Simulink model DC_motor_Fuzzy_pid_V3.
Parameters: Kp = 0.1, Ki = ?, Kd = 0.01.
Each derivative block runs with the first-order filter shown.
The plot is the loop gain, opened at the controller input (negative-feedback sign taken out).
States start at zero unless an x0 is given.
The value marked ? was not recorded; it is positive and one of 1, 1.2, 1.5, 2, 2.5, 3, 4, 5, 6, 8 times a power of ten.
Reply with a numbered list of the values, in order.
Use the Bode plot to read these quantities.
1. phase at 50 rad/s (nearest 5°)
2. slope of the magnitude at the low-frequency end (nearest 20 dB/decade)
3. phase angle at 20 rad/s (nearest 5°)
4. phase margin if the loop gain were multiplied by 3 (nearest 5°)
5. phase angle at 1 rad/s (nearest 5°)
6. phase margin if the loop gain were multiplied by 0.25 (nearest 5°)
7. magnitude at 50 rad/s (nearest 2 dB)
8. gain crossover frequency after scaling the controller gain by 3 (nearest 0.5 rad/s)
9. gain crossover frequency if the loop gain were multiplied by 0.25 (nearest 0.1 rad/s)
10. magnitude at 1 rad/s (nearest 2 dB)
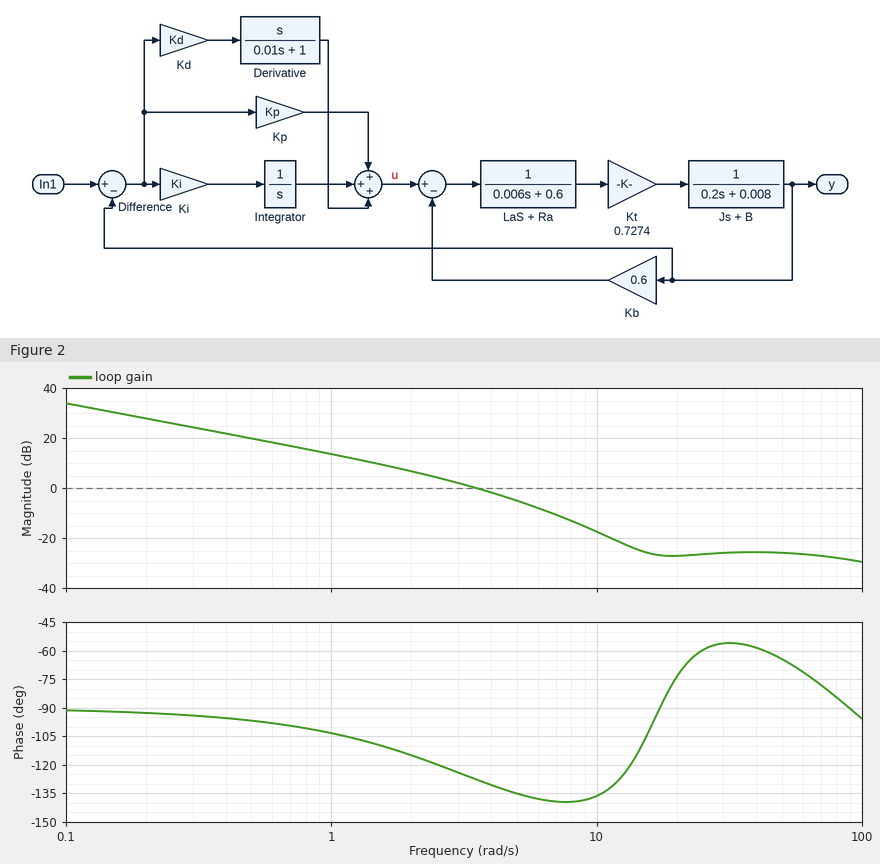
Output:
1. -65°
2. -20 dB/decade
3. -75°
4. 40°
5. -105°
6. 75°
7. -26 dB
8. 6.5 rad/s
9. 1.2 rad/s
10. 14 dB
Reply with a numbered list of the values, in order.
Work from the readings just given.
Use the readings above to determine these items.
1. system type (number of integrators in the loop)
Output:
1. 1
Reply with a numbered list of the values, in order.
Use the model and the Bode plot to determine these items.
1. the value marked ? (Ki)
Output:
1. 3
